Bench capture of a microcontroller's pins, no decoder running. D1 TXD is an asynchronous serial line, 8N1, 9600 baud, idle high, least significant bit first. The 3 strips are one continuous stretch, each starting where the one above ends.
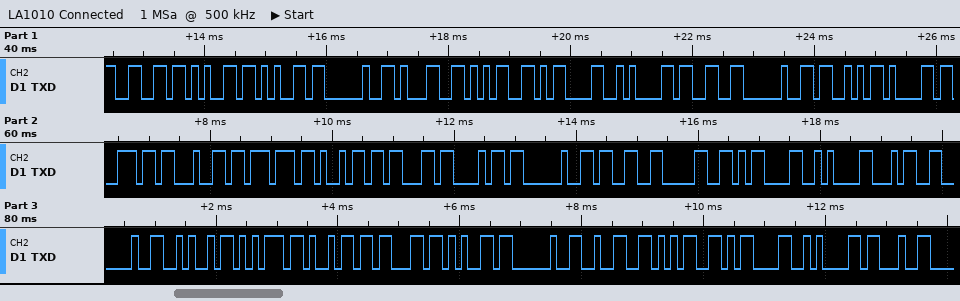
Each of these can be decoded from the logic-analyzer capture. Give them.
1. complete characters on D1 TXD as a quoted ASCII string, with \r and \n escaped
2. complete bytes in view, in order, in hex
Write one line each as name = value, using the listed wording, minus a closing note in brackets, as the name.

complete characters on D1 TXD as a quoted ASCII string, with \r and \n escaped = "fee 15\r\n3 Sandwich 30\r\n4 Juice 25\r\n#"
complete bytes in view, in order, in hex = 66 65 65 20 31 35 0D 0A 33 20 53 61 6E 64 77 69 63 68 20 33 30 0D 0A 34 20 4A 75 69 63 65 20 32 35 0D 0A 23
